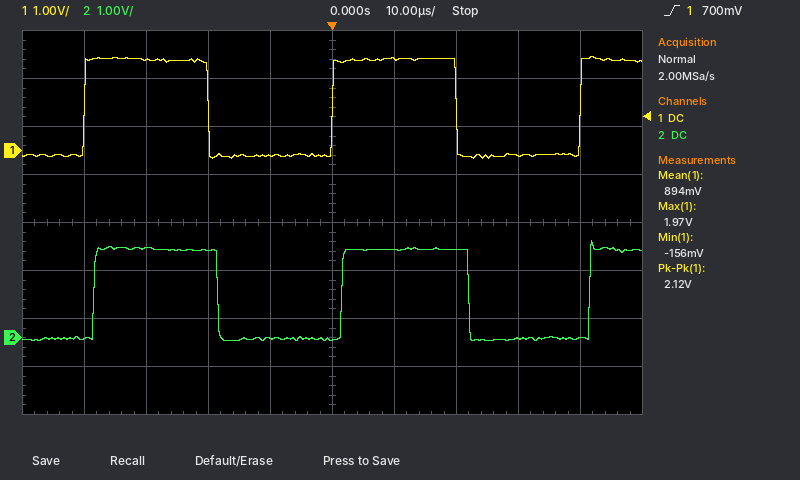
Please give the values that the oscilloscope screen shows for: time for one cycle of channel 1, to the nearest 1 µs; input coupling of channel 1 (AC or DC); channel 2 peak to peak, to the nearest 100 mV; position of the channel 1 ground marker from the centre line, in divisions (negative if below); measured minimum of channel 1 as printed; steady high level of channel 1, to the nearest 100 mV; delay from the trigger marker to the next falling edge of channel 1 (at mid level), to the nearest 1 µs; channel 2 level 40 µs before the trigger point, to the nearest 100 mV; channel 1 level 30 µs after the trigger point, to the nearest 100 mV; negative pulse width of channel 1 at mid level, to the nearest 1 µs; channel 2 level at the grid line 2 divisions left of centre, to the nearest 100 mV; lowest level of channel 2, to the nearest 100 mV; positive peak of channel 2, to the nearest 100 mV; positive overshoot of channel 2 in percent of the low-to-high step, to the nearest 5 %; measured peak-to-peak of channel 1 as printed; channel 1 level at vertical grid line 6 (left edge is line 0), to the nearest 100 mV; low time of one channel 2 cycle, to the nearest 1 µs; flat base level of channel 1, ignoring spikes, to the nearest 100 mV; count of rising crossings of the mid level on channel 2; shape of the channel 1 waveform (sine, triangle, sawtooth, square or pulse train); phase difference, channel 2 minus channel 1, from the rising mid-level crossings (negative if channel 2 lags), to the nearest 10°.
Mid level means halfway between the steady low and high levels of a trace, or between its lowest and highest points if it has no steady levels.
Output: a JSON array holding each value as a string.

["40 µs", "DC", "2.1 V", "+1.5 div", "-156 mV", "1.9 V", "20 µs", "0.0 V", "-100 mV", "20 µs", "1.8 V", "-100 mV", "2.0 V", "10 %", "2.12 V", "1.9 V", "20 µs", "-100 mV", "3", "square", "-10°"]
